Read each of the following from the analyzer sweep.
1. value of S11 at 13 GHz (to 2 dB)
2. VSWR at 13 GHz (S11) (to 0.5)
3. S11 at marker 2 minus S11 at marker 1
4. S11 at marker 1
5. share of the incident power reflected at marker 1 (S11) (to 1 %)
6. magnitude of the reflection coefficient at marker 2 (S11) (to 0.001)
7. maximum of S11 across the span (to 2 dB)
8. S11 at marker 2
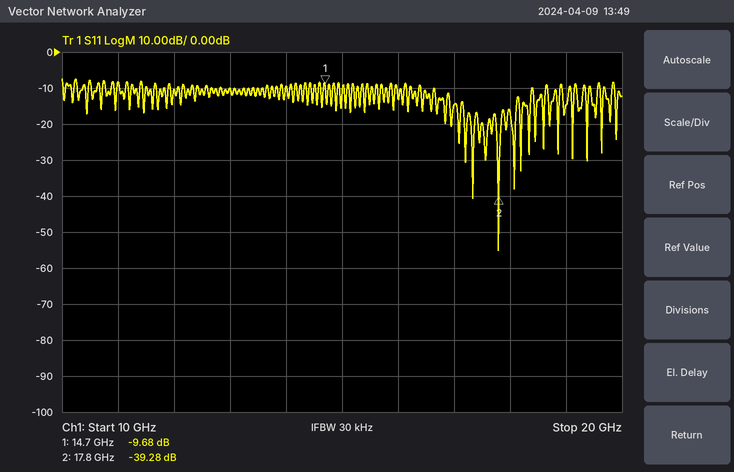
-10 dB
2.0
-29.60 dB
-9.68 dB
11 %
0.011
-8 dB
-39.28 dB
